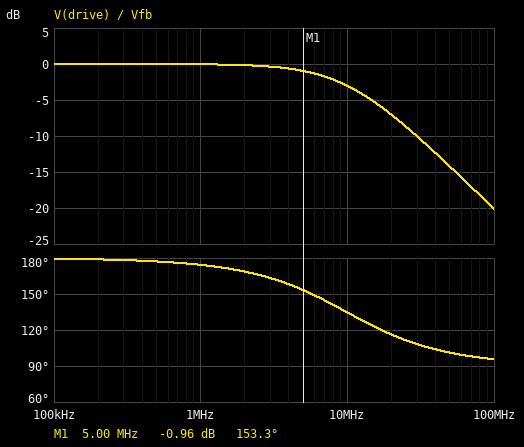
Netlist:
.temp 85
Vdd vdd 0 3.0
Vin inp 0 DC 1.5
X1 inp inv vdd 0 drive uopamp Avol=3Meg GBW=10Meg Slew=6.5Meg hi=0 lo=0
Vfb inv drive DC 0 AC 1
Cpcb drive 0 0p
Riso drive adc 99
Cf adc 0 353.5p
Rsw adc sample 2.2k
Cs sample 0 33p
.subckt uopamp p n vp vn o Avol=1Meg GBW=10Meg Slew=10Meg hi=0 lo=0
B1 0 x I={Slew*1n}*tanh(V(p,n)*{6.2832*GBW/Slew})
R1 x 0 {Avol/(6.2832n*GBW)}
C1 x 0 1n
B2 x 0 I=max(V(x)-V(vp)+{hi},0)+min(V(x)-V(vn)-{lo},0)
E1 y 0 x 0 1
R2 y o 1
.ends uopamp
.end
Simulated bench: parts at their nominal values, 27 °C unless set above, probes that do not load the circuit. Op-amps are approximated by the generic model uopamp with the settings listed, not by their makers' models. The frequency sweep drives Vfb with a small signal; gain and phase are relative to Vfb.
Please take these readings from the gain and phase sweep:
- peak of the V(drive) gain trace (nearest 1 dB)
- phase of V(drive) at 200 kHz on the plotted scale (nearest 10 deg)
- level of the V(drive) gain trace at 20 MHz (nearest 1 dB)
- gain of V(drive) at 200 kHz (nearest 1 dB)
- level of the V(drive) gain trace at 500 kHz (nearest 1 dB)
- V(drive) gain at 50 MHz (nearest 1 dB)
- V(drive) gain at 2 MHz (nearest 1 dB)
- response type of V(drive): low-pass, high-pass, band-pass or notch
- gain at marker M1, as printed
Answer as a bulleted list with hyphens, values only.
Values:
- 0 dB
- 180 deg
- -7 dB
- 0 dB
- 0 dB
- -14 dB
- 0 dB
- low-pass
- -0.96 dB
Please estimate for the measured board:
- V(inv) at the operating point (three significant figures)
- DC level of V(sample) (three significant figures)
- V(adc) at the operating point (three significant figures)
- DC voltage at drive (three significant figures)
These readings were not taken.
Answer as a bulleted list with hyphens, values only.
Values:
- 1.50 V
- 1.50 V
- 1.50 V
- 1.50 V
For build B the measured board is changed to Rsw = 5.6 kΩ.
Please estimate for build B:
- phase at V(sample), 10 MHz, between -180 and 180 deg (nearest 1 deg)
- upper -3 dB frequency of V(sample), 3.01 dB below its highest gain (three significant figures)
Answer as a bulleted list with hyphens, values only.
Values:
- -16 deg
- 812 kHz
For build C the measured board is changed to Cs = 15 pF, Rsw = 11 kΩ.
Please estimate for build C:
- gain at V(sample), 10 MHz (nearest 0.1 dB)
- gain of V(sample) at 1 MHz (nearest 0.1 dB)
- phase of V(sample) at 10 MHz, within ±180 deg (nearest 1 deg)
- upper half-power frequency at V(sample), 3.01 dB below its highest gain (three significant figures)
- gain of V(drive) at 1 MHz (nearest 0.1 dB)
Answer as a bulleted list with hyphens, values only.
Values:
- -31.1 dB
- -3.5 dB
- -15 deg
- 910 kHz
- 0 dB
